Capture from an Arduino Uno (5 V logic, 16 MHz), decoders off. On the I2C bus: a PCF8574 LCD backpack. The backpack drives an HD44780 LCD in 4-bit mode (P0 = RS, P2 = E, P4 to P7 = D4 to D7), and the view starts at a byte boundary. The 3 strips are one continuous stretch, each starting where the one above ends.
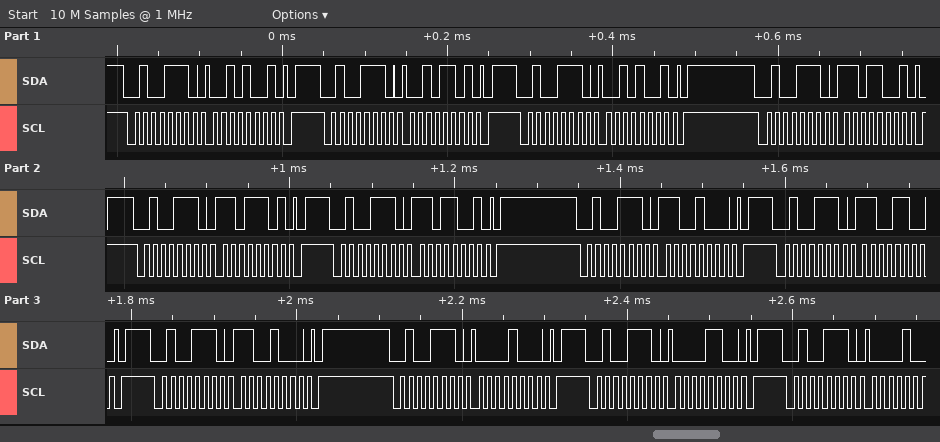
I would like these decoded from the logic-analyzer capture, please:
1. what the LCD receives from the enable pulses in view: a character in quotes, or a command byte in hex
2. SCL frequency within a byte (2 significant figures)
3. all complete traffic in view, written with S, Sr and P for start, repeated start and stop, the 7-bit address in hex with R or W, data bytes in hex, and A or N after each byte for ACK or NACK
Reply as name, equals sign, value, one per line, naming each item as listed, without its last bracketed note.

what the LCD receives from the enable pulses in view: a character in quotes, or a command byte in hex = '-'
SCL frequency within a byte = 100 kHz
all complete traffic in view, written with S, Sr and P for start, repeated start and stop, the 7-bit address in hex with R or W, data bytes in hex, and A or N after each byte for ACK or NACK = S 27W A 29 A P S 27W A 2D A P S 27W A 29 A P S 27W A D9 A P S 27W A DD A P S 27W A D9 A P S 27W A C8 A P S 27W A CC A P S 27W A C8 A P S 27W A 08 A P S 27W A 0C A P S 27W A
